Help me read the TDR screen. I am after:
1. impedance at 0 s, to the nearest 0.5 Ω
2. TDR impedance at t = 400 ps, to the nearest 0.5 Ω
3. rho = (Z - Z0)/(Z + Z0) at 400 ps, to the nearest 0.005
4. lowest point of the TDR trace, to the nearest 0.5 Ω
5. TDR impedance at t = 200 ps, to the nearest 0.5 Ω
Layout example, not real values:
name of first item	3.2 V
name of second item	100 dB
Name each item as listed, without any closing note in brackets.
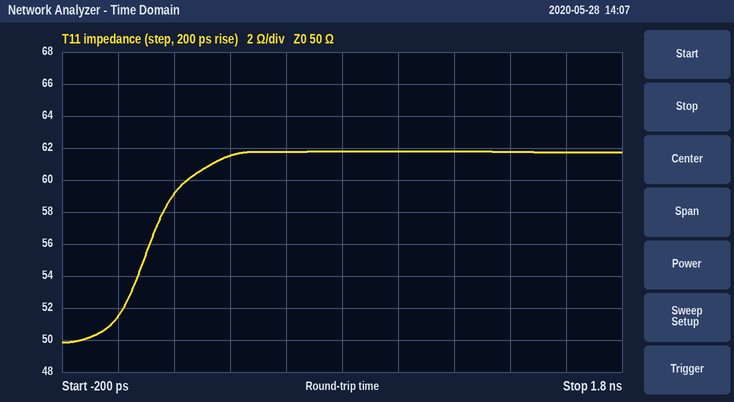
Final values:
impedance at 0 s, to the nearest 0.5 Ω	51.5 Ω
TDR impedance at t = 400 ps, to the nearest 0.5 Ω	61.5 Ω
rho = (Z - Z0)/(Z + Z0) at 400 ps, to the nearest 0.005	+0.105
lowest point of the TDR trace, to the nearest 0.5 Ω	50.0 Ω
TDR impedance at t = 200 ps, to the nearest 0.5 Ω	59.0 Ω
